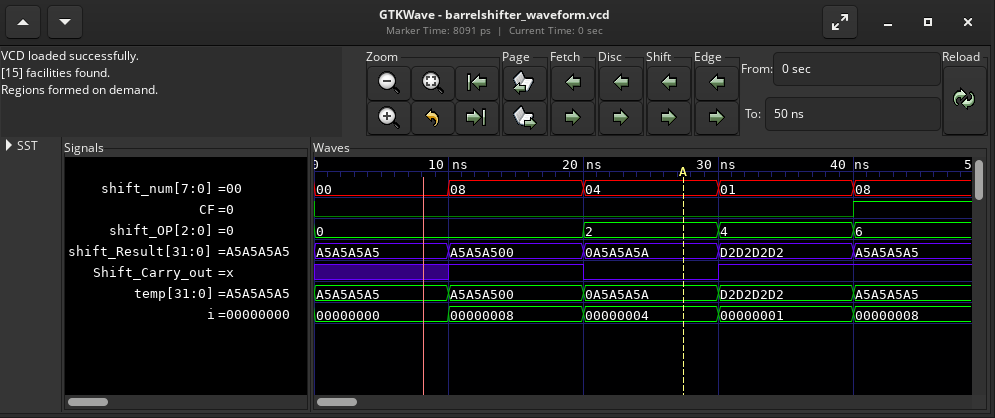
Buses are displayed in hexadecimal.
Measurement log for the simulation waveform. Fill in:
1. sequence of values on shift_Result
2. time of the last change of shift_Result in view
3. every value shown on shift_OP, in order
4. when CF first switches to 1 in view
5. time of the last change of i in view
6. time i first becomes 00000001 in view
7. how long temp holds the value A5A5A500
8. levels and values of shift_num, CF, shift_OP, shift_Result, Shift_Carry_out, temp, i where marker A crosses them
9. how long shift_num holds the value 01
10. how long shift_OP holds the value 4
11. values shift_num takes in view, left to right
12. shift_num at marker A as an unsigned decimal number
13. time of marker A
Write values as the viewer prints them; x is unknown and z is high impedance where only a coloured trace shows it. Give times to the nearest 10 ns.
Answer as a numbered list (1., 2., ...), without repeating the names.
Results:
1. A5A5A5A5, A5A5A500, 0A5A5A5A, D2D2D2D2, A5A5A5A5
2. 40 ns
3. 0, 2, 4, 6
4. 40 ns
5. 40 ns
6. 30 ns
7. 10 ns
8. shift_num=04, CF=0, shift_OP=2, shift_Result=0A5A5A5A, Shift_Carry_out=0, temp=0A5A5A5A, i=00000004
9. 10 ns
10. 10 ns
11. 00, 08, 04, 01, 08
12. 4
13. 30 ns
